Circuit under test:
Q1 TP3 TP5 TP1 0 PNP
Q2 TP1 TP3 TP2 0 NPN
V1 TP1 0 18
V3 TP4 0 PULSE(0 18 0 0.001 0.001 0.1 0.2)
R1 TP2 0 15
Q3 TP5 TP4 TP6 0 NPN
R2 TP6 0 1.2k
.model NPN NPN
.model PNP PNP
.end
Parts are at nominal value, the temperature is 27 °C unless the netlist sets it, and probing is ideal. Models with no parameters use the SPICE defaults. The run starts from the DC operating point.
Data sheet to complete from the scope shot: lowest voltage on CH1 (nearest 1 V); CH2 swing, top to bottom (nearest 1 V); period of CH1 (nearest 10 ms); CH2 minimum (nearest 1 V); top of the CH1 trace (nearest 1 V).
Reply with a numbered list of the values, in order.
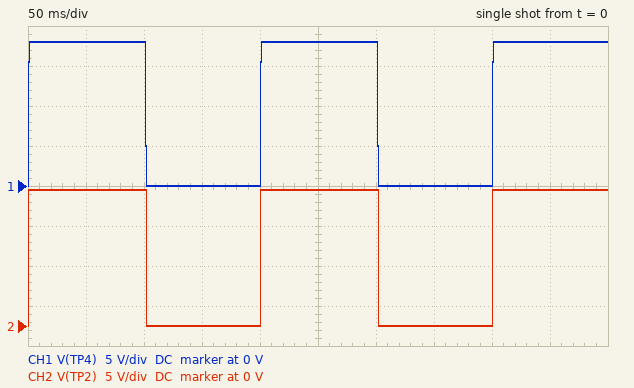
1. 0 V
2. 17 V
3. 200 ms
4. 0 V
5. 18 V
